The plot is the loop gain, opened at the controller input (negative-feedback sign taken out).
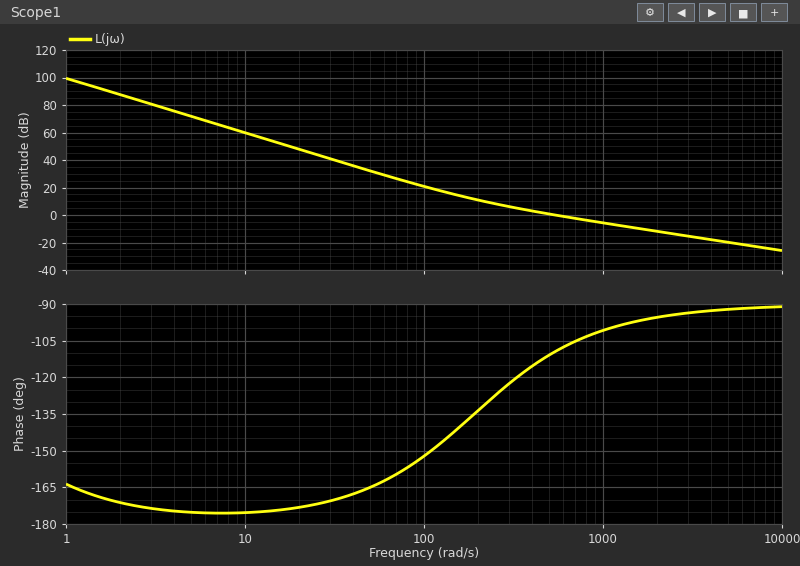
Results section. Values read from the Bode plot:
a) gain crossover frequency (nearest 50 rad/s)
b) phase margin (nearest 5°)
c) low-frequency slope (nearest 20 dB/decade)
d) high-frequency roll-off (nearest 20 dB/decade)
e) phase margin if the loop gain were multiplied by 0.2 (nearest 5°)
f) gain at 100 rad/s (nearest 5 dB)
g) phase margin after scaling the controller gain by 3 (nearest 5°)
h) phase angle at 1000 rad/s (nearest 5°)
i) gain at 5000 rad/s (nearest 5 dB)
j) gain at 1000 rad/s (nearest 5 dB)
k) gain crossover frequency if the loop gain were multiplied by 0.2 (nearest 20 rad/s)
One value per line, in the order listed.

550 rad/s
70°
-40 dB/decade
-20 dB/decade
40°
20 dB
85°
-100°
-20 dB
-5 dB
160 rad/s
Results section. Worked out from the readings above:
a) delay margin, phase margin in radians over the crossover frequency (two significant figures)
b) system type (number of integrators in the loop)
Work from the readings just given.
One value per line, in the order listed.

0.0022 s
2
